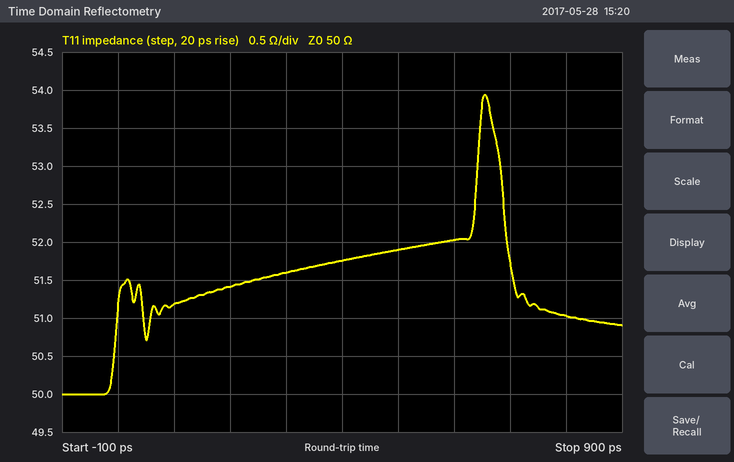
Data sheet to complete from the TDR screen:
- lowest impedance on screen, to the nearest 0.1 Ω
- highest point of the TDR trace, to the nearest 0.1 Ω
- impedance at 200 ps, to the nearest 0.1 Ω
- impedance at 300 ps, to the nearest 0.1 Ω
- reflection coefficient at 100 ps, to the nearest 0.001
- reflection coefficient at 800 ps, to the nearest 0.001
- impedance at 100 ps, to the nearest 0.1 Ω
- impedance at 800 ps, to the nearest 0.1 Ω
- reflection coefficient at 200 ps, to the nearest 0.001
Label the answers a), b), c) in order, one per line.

a) 50.0 Ω
b) 53.9 Ω
c) 51.4 Ω
d) 51.6 Ω
e) +0.012
f) +0.010
g) 51.2 Ω
h) 51.0 Ω
i) +0.014
